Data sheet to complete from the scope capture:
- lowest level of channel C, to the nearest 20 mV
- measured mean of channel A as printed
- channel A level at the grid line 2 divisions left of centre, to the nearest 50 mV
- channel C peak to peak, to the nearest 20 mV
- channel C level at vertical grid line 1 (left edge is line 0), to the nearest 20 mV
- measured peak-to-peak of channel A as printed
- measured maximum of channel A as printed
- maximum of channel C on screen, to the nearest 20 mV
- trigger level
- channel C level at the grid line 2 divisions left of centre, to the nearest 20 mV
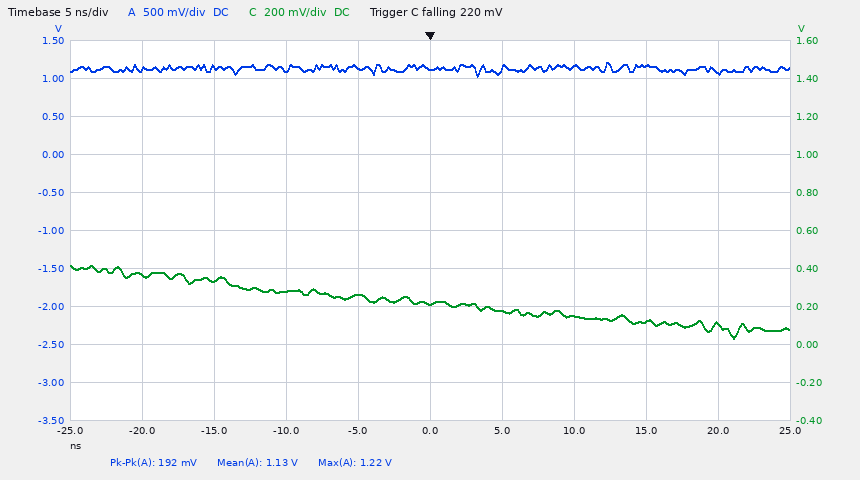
40 mV
1.13 V
1.10 V
380 mV
360 mV
192 mV
1.22 V
420 mV
220 mV
280 mV
